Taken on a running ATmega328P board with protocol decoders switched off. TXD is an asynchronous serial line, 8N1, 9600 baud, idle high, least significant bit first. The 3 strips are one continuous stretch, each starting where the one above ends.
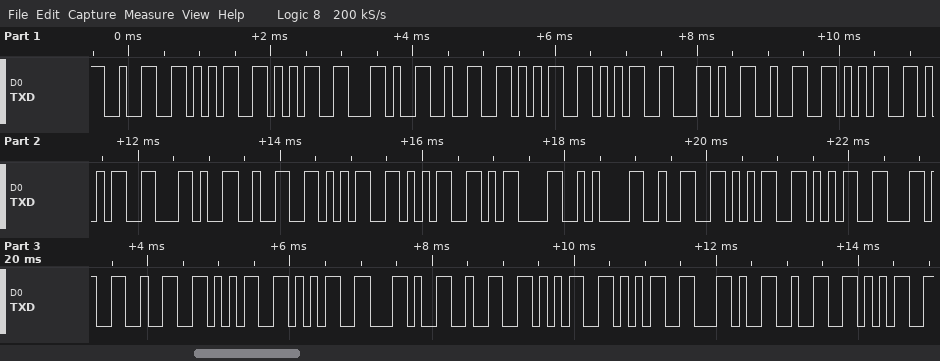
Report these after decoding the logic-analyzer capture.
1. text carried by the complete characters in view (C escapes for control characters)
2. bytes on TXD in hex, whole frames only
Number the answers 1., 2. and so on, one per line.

1. "255,255,255,255\r\n255,255,255,25"
2. 32 35 35 2C 32 35 35 2C 32 35 35 2C 32 35 35 0D 0A 32 35 35 2C 32 35 35 2C 32 35 35 2C 32 35
